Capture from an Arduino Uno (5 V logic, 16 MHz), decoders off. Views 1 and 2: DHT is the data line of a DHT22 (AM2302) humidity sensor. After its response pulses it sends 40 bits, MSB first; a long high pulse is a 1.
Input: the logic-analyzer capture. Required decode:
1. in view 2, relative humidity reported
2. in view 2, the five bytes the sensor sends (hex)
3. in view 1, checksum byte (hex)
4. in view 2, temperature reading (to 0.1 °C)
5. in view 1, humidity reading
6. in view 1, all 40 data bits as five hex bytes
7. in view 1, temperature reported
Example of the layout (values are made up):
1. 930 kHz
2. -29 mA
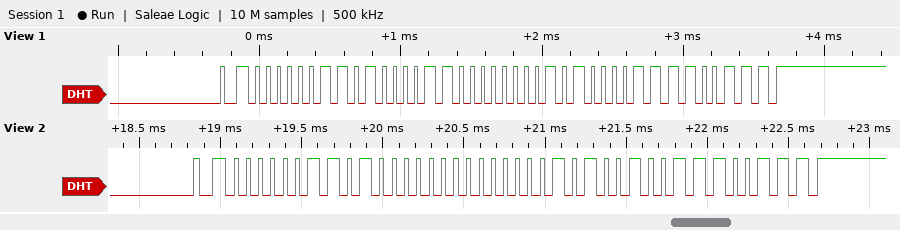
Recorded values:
1. 83.2 %
2. 03 40 00 A4 E7
3. 0xE7
4. 16.4 °C
5. 83.5 %
6. 03 43 00 A1 E7
7. 16.1 °C
